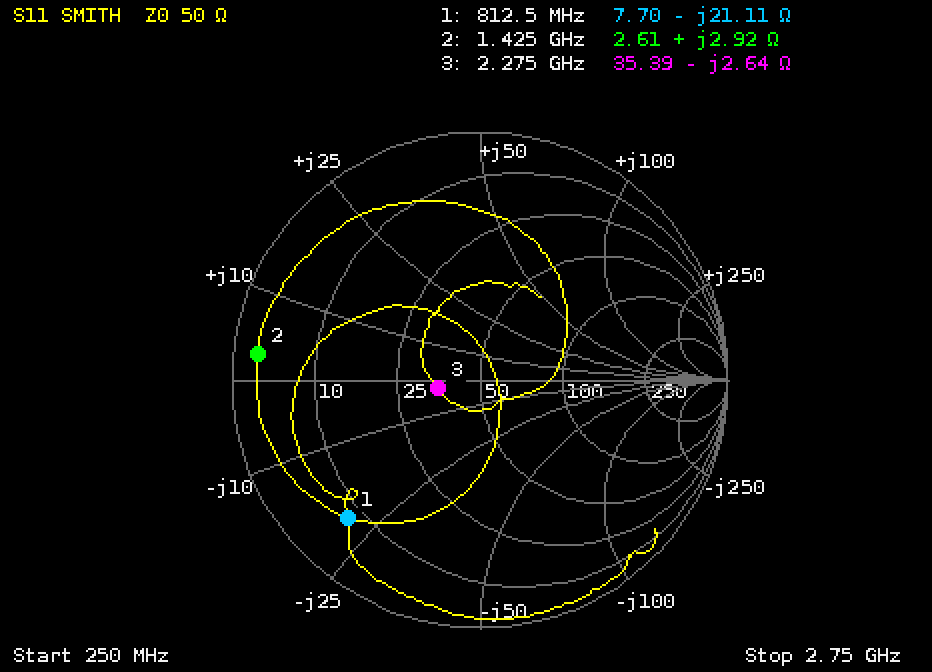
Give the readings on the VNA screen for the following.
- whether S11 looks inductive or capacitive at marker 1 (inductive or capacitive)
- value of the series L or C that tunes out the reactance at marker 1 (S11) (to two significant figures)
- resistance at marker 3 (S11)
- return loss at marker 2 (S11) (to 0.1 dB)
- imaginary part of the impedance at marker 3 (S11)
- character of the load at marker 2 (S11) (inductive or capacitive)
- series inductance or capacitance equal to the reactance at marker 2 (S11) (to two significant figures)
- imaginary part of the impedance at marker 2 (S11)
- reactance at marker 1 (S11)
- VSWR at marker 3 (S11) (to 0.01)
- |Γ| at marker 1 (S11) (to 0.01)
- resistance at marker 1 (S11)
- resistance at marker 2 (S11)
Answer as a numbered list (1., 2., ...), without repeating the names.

1. capacitive
2. 4.1 nH
3. 35.39 Ω
4. 0.9 dB
5. -2.64 Ω
6. inductive
7. 330 pH
8. +2.92 Ω
9. -21.11 Ω
10. 1.42
11. 0.77
12. 7.70 Ω
13. 2.61 Ω
